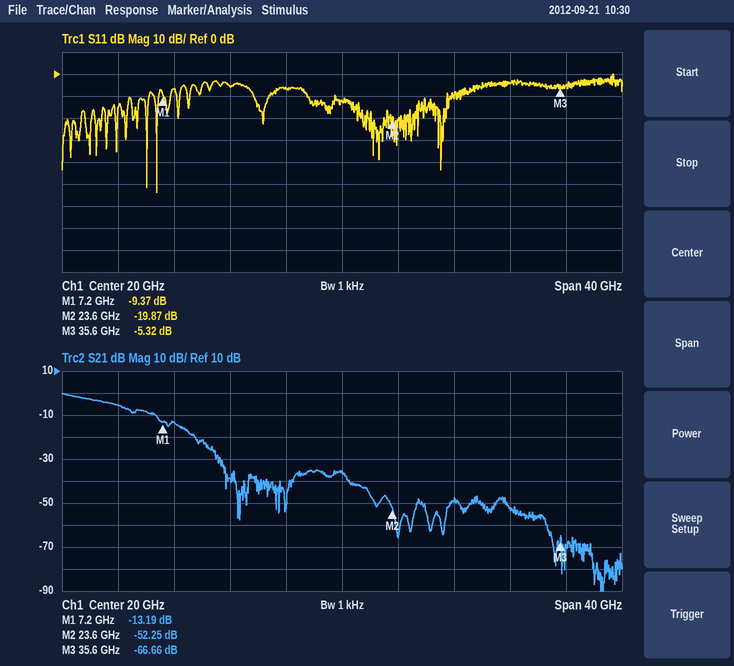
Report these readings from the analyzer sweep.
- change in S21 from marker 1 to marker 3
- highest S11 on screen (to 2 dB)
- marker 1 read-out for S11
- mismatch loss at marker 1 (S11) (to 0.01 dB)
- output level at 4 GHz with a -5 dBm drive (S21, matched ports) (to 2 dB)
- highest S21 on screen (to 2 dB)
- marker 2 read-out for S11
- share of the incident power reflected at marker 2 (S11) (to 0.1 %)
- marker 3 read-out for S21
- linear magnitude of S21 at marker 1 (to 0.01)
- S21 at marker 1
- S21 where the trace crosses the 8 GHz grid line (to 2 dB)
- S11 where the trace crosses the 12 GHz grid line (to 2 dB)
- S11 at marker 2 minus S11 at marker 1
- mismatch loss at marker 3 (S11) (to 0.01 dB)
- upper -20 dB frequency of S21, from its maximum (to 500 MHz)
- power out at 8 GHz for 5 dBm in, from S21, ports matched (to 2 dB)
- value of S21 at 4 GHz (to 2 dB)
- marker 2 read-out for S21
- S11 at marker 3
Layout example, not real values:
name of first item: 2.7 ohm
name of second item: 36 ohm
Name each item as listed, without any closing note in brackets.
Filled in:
change in S21 from marker 1 to marker 3: -53.47 dB
highest S11 on screen: 0 dB
marker 1 read-out for S11: -9.37 dB
mismatch loss at marker 1 (S11): 0.53 dB
output level at 4 GHz with a -5 dBm drive (S21, matched ports): -10 dBm
highest S21 on screen: 0 dB
marker 2 read-out for S11: -19.87 dB
share of the incident power reflected at marker 2 (S11): 1.0 %
marker 3 read-out for S21: -66.66 dB
linear magnitude of S21 at marker 1: 0.22
S21 at marker 1: -13.19 dB
S21 where the trace crosses the 8 GHz grid line: -14 dB
S11 where the trace crosses the 12 GHz grid line: -6 dB
S11 at marker 2 minus S11 at marker 1: -10.50 dB
mismatch loss at marker 3 (S11): 1.51 dB
upper -20 dB frequency of S21, from its maximum: 9.5 GHz
power out at 8 GHz for 5 dBm in, from S21, ports matched: -8 dBm
value of S21 at 4 GHz: -6 dB
marker 2 read-out for S21: -52.25 dB
S11 at marker 3: -5.32 dB
